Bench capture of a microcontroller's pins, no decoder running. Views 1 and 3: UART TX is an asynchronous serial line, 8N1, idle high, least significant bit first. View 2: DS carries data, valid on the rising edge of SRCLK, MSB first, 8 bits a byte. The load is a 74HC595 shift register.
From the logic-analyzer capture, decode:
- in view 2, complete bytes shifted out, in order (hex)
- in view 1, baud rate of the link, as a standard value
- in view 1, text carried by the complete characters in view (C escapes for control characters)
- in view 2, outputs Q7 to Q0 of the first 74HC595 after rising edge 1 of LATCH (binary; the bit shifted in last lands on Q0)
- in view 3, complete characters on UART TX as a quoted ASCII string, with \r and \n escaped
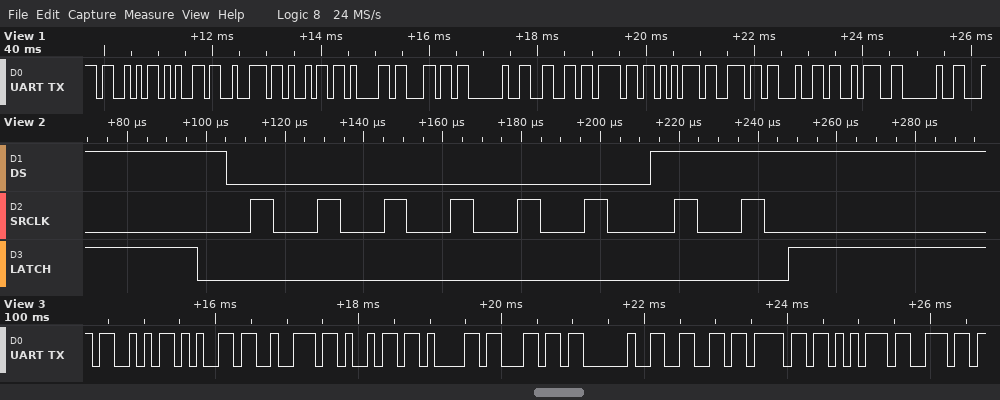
0x03
9600 baud
"Serial found: "
00000011
"Serial foun"
